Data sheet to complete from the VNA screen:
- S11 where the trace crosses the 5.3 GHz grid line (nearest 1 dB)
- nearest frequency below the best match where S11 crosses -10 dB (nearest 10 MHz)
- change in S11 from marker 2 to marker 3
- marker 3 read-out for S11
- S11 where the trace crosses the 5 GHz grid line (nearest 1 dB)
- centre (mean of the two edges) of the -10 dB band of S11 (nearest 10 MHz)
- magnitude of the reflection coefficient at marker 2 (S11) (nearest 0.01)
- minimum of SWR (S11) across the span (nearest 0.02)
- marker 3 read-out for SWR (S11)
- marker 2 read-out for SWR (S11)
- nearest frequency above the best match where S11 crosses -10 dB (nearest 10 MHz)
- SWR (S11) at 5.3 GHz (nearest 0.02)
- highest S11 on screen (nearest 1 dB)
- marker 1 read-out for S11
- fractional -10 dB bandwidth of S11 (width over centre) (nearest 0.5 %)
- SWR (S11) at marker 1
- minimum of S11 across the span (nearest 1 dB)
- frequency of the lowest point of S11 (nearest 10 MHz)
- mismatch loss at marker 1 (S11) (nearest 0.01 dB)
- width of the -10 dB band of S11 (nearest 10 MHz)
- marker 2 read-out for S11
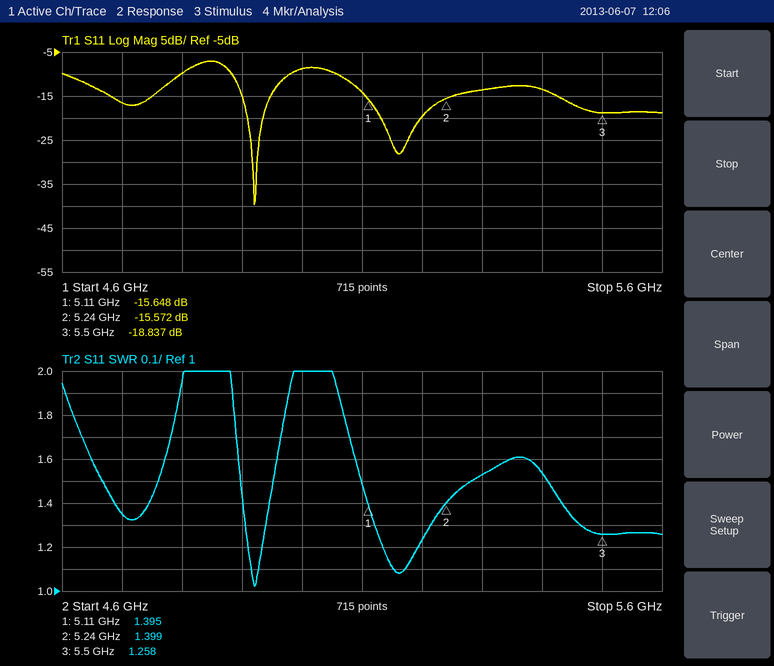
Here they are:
-14 dB
4.88 GHz
-3.265 dB
-18.837 dB
-9 dB
4.93 GHz
0.17
1.02
1.258
1.399
4.98 GHz
1.52
-7 dB
-15.648 dB
2.0 %
1.395
-40 dB
4.92 GHz
0.12 dB
100 MHz
-15.572 dB
